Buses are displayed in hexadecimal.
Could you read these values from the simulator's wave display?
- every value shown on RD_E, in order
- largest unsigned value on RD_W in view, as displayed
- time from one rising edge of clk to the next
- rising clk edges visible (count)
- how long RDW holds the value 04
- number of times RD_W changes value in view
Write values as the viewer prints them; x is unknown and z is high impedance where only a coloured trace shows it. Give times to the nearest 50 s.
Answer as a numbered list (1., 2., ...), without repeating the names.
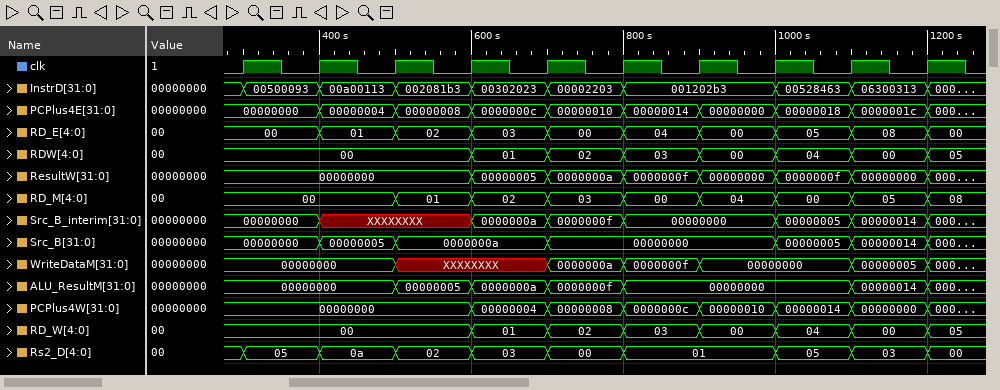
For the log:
1. 00, 01, 02, 03, 00, 04, 00, 05, 08, 00
2. 05
3. 100 s
4. 10
5. 100 s
6. 7
